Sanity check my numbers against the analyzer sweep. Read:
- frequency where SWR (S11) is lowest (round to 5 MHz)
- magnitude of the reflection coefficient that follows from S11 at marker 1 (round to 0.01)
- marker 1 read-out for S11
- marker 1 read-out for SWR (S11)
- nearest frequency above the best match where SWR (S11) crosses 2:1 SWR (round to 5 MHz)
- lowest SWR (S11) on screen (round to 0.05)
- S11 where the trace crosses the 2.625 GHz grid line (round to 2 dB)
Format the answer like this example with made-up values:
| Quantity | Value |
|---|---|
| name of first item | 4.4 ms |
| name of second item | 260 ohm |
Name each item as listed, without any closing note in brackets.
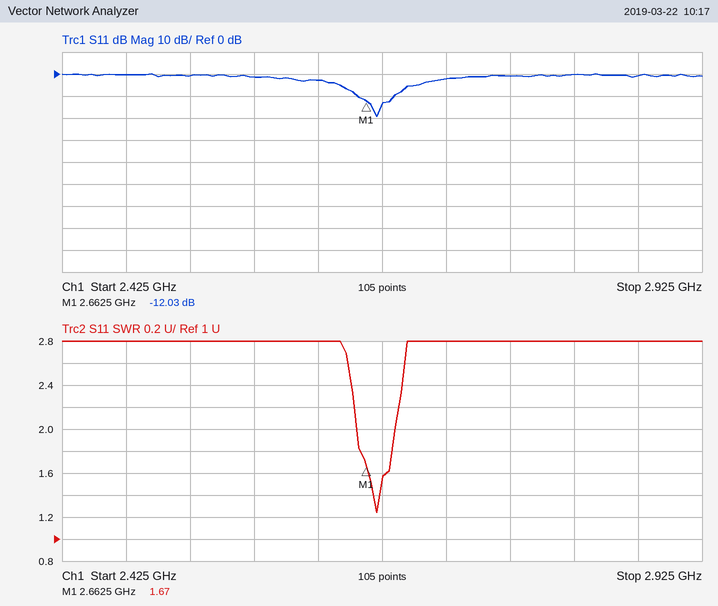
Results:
| Quantity | Value |
|---|---|
| frequency where SWR (S11) is lowest | 2.670 GHz |
| magnitude of the reflection coefficient that follows from S11 at marker 1 | 0.25 |
| marker 1 read-out for S11 | -12.03 dB |
| marker 1 read-out for SWR | 1.67 |
| nearest frequency above the best match where SWR (S11) crosses 2:1 SWR | 2.685 GHz |
| lowest SWR (S11) on screen | 1.25 |
| S11 where the trace crosses the 2.625 GHz grid line | -2 dB |
